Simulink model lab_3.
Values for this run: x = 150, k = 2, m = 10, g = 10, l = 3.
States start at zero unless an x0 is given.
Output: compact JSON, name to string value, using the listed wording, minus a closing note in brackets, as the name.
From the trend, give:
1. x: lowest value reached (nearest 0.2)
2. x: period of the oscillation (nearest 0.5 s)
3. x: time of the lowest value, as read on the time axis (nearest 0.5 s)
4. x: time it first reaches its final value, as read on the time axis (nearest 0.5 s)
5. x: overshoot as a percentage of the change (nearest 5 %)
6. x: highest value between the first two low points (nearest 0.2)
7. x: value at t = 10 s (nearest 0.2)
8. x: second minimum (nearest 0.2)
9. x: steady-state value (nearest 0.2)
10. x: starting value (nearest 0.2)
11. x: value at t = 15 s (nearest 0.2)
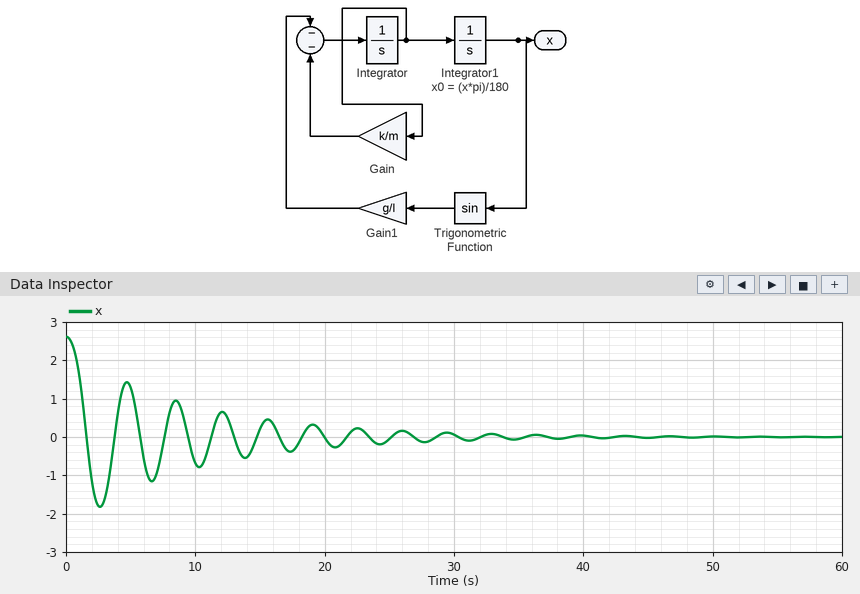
{"x: lowest value reached": "-1.8", "x: period of the oscillation": "4.0 s", "x: time of the lowest value, as read on the time axis": "2.5 s", "x: time it first reaches its final value, as read on the time axis": "1.5 s", "x: overshoot as a percentage of the change": "70 %", "x: highest value between the first two low points": "1.4", "x: value at t = 10 s": "-0.6", "x: second minimum": "-1.2", "x: steady-state value": "0.0", "x: starting value": "2.6", "x: value at t = 15 s": "0.2"}
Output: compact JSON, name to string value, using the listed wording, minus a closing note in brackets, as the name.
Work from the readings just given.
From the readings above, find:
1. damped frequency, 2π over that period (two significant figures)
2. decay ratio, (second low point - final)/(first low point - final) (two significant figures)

{"damped frequency, 2π over that period": "1.6 rad/s", "decay ratio, (second low point - final)/(first low point - final)": "0.67"}
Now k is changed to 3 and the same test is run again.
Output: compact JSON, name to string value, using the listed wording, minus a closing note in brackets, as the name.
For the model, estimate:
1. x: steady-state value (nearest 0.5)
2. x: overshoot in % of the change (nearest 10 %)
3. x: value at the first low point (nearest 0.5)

{"x: steady-state value": "0.0", "x: overshoot in % of the change": "60 %", "x: value at the first low point": "-1.5"}
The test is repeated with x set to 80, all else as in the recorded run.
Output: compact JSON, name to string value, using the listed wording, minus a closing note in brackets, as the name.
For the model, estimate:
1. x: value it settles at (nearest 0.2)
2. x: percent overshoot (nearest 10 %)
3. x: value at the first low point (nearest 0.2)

{"x: value it settles at": "0.0", "x: percent overshoot": "80 %", "x: value at the first low point": "-1.2"}
